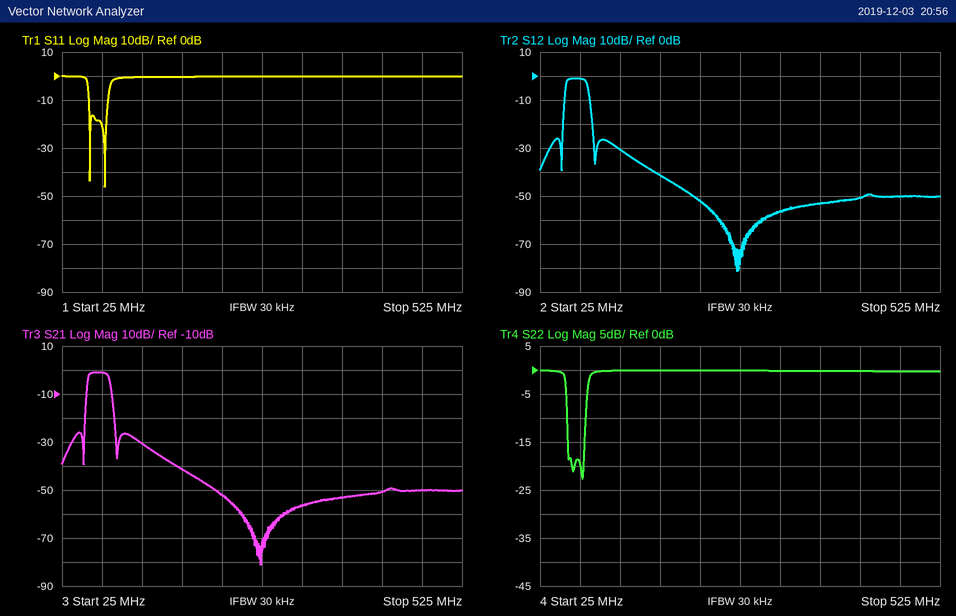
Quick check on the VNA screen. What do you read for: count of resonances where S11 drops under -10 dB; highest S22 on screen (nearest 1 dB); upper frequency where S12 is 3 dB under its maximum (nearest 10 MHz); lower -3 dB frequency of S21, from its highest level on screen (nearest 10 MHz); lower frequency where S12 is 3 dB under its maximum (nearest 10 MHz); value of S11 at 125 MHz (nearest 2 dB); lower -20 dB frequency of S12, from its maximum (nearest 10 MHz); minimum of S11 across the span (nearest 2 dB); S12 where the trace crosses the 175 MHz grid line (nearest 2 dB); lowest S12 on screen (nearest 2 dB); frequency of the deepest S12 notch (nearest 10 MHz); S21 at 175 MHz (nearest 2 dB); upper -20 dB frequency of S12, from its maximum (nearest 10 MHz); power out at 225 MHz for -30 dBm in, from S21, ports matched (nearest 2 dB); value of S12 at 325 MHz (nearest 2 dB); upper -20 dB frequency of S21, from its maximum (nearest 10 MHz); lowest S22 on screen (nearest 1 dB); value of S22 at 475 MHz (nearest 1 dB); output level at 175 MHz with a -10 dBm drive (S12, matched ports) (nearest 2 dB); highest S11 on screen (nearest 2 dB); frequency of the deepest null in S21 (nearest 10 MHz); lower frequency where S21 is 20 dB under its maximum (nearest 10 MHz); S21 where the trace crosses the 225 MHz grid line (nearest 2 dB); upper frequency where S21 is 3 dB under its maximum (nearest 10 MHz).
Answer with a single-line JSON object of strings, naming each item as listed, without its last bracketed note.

{"count of resonances where S11 drops under -10 dB": "2", "highest S22 on screen": "0 dB", "upper frequency where S12 is 3 dB under its maximum": "80 MHz", "lower -3 dB frequency of S21, from its highest level on screen": "60 MHz", "lower frequency where S12 is 3 dB under its maximum": "60 MHz", "value of S11 at 125 MHz": "0 dB", "lower -20 dB frequency of S12, from its maximum": "50 MHz", "minimum of S11 across the span": "-46 dB", "S12 where the trace crosses the 175 MHz grid line": "-42 dB", "lowest S12 on screen": "-82 dB", "frequency of the deepest S12 notch": "270 MHz", "S21 at 175 MHz": "-42 dB", "upper -20 dB frequency of S12, from its maximum": "90 MHz", "power out at 225 MHz for -30 dBm in, from S21, ports matched": "-82 dBm", "value of S12 at 325 MHz": "-56 dB", "upper -20 dB frequency of S21, from its maximum": "90 MHz", "lowest S22 on screen": "-23 dB", "value of S22 at 475 MHz": "0 dB", "output level at 175 MHz with a -10 dBm drive (S12, matched ports)": "-52 dBm", "highest S11 on screen": "0 dB", "frequency of the deepest null in S21": "270 MHz", "lower frequency where S21 is 20 dB under its maximum": "50 MHz", "S21 where the trace crosses the 225 MHz grid line": "-52 dB", "upper frequency where S21 is 3 dB under its maximum": "80 MHz"}
